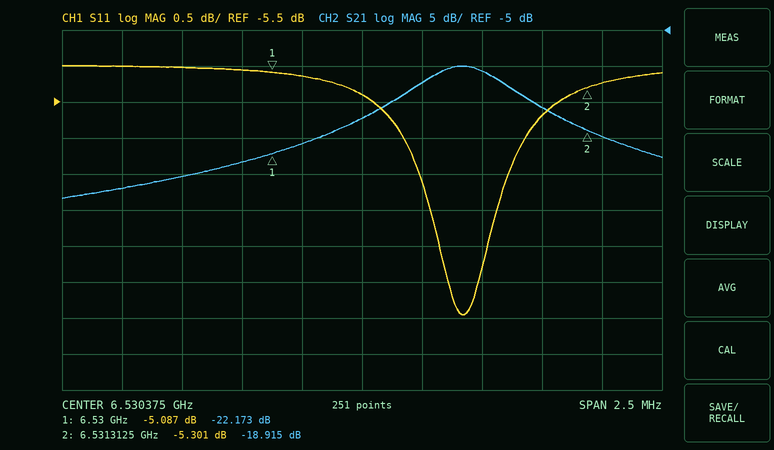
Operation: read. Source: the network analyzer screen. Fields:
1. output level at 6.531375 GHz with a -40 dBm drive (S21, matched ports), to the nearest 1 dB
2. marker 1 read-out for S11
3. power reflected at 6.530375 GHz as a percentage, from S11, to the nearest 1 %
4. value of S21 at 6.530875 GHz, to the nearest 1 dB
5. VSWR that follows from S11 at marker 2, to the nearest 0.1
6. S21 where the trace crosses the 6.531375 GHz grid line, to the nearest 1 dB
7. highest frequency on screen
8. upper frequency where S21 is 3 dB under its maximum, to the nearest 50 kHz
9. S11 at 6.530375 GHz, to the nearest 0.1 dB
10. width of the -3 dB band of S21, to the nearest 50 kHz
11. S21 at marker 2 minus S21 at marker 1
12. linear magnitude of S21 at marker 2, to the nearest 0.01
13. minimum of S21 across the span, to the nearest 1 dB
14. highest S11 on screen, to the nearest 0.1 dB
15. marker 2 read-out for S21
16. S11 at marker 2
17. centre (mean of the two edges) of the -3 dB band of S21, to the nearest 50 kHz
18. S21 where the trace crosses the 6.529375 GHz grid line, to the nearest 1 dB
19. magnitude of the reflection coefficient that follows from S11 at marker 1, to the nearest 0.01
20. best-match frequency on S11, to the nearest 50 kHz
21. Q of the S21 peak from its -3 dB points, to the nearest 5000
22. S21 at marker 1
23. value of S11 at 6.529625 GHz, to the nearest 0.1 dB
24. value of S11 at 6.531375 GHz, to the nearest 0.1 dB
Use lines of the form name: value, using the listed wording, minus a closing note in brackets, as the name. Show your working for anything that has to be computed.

output level at 6.531375 GHz with a -40 dBm drive (S21, matched ports), to the nearest 1 dB: -40 dBm + (-20 dB) = -60 dBm
marker 1 read-out for S11: -5.087 dB
power reflected at 6.530375 GHz as a percentage, from S11, to the nearest 1 %: 10^(-5.4/10) ≈ 29 %
value of S21 at 6.530875 GHz, to the nearest 1 dB: -11 dB
VSWR that follows from S11 at marker 2, to the nearest 0.1: (1 + 0.5432)/(1 − 0.5432) ≈ 3.4
S21 where the trace crosses the 6.531375 GHz grid line, to the nearest 1 dB: -20 dB
highest frequency on screen: 6.531625 GHz
upper frequency where S21 is 3 dB under its maximum, to the nearest 50 kHz: 6.53100 GHz
S11 at 6.530375 GHz, to the nearest 0.1 dB: -5.4 dB
width of the -3 dB band of S21, to the nearest 50 kHz: 6.53100 GHz − 6.53060 GHz = 400 kHz
S21 at marker 2 minus S21 at marker 1: -18.915 − (-22.173) = 3.258 dB
linear magnitude of S21 at marker 2, to the nearest 0.01: 10^(-18.915/20) ≈ 0.11
minimum of S21 across the span, to the nearest 1 dB: -28 dB
highest S11 on screen, to the nearest 0.1 dB: -5.0 dB
marker 2 read-out for S21: -18.915 dB
S11 at marker 2: -5.301 dB
centre (mean of the two edges) of the -3 dB band of S21, to the nearest 50 kHz: 6.53080 GHz
S21 where the trace crosses the 6.529375 GHz grid line, to the nearest 1 dB: -27 dB
magnitude of the reflection coefficient that follows from S11 at marker 1, to the nearest 0.01: 10^(-5.087/20) ≈ 0.56
best-match frequency on S11, to the nearest 50 kHz: 6.53080 GHz
Q of the S21 peak from its -3 dB points, to the nearest 5000: 6.5308 GHz / 400 kHz ≈ 16327, so 15000 to the nearest 5000
S21 at marker 1: -22.173 dB
value of S11 at 6.529625 GHz, to the nearest 0.1 dB: -5.0 dB
value of S11 at 6.531375 GHz, to the nearest 0.1 dB: -5.2 dB
